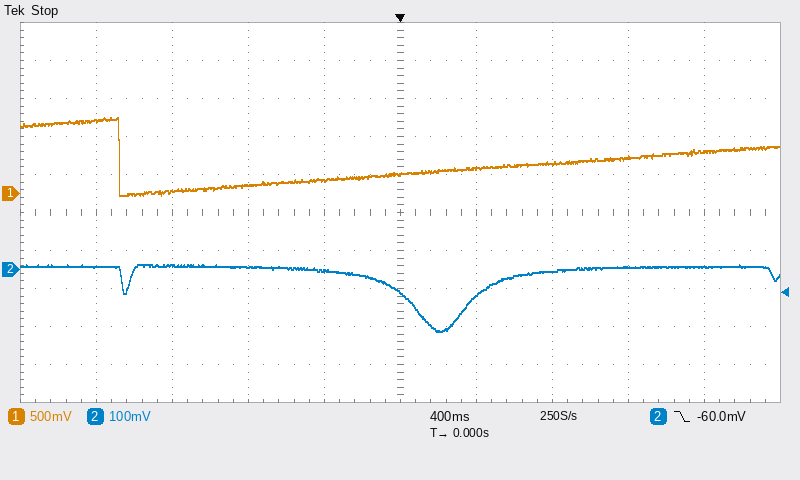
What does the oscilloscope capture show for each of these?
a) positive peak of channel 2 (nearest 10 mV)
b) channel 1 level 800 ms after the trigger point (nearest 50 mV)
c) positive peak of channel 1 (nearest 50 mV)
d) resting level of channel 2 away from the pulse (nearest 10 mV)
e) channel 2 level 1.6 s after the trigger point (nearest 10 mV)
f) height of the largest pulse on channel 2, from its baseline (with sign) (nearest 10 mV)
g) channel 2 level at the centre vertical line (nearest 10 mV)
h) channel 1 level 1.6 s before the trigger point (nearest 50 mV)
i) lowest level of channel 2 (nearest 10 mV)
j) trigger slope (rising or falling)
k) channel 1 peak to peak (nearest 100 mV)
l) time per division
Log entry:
10 mV
400 mV
1.00 V
10 mV
10 mV
-170 mV
-60 mV
950 mV
-160 mV
falling
1.00 V
400 ms
